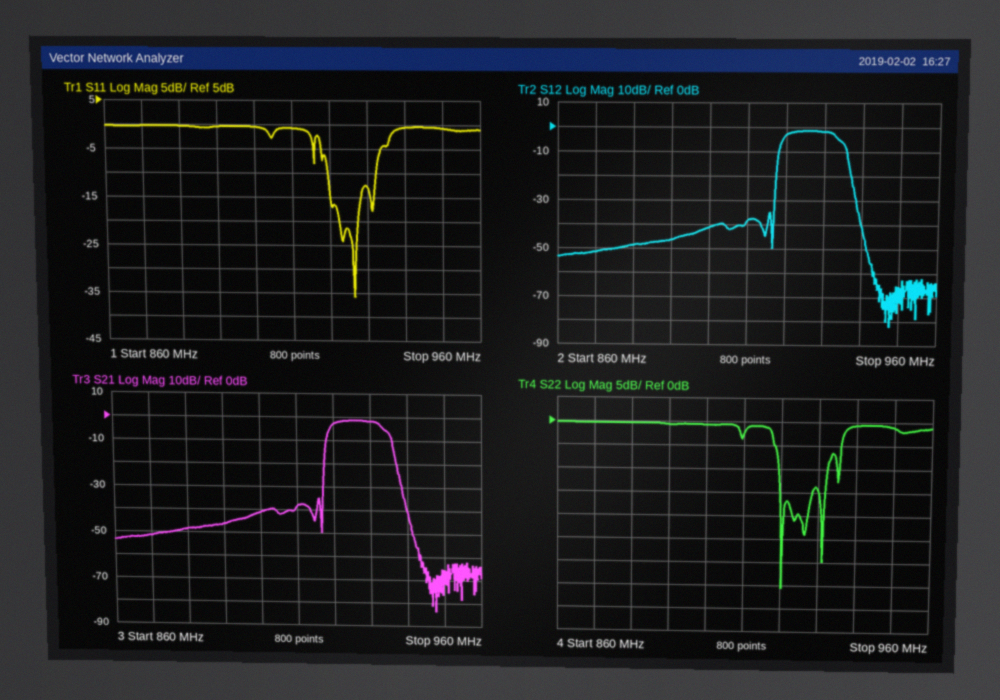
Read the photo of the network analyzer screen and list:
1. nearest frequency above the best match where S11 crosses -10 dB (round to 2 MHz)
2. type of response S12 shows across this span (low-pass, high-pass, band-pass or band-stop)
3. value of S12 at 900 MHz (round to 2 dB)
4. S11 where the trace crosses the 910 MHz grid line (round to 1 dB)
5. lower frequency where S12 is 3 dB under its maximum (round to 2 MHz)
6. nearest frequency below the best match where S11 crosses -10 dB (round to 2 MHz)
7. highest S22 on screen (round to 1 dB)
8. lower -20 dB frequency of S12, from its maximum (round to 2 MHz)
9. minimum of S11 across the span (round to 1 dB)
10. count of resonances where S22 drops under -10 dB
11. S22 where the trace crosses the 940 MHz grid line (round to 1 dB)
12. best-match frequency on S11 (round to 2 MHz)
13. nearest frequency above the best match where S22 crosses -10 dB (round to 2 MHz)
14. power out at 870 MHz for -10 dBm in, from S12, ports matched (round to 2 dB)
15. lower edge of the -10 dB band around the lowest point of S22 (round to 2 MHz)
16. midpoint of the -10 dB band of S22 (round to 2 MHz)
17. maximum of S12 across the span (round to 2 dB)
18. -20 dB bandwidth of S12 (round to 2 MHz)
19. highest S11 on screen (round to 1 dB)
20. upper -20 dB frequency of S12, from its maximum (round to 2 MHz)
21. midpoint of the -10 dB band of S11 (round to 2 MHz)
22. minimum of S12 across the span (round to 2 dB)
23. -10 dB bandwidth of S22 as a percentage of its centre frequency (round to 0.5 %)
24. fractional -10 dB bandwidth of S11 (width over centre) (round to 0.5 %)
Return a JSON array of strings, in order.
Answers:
["932 MHz", "band-pass", "-42 dB", "-1 dB", "920 MHz", "920 MHz", "0 dB", "918 MHz", "-36 dB", "4", "-1 dB", "926 MHz", "932 MHz", "-62 dBm", "920 MHz", "926 MHz", "-2 dB", "20 MHz", "0 dB", "938 MHz", "926 MHz", "-82 dB", "1.5 %", "1.5 %"]
